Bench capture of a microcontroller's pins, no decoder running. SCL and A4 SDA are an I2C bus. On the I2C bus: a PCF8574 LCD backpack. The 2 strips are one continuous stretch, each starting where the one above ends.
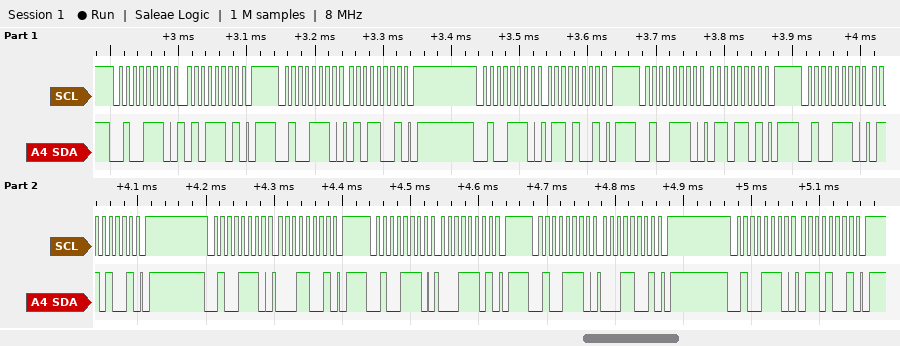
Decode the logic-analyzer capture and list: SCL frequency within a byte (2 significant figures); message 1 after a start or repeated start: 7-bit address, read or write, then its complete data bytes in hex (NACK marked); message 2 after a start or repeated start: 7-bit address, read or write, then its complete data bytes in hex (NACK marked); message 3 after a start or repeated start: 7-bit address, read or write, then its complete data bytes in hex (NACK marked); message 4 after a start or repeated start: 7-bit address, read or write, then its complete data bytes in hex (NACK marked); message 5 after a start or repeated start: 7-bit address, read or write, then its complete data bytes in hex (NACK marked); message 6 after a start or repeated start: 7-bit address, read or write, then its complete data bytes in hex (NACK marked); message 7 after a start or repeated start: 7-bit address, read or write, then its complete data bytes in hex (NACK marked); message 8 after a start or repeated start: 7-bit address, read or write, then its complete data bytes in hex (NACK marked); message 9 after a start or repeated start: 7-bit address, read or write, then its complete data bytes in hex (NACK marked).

100 kHz
0x27 write: 5D
0x27 write: 59
0x27 write: 69
0x27 write: 6D
0x27 write: 69
0x27 write: 19
0x27 write: 1D
0x27 write: 19
0x27 write: 69
